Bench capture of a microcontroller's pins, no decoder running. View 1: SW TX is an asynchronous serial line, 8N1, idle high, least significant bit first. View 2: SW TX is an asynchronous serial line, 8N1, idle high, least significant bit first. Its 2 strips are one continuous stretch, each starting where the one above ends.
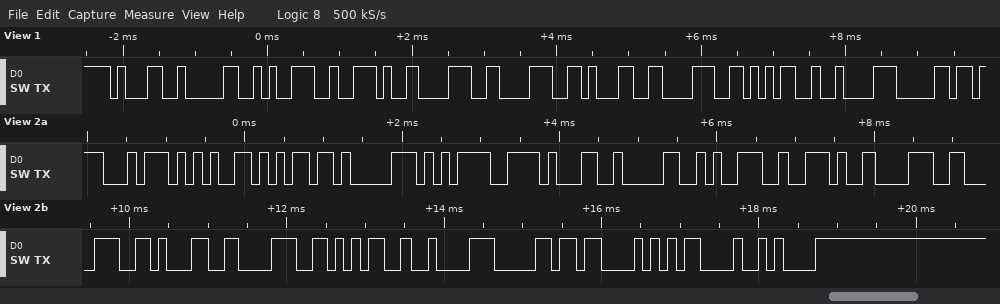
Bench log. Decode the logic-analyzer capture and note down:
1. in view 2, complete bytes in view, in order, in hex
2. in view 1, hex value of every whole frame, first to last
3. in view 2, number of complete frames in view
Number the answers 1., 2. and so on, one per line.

1. 74 65 6D 70 3D 31 30 39 2E 38 38 31 38 35 C2 B0 43 0D 0A
2. 31 30 39 2E 38 38 31 38 35 C2 B0
3. 19
